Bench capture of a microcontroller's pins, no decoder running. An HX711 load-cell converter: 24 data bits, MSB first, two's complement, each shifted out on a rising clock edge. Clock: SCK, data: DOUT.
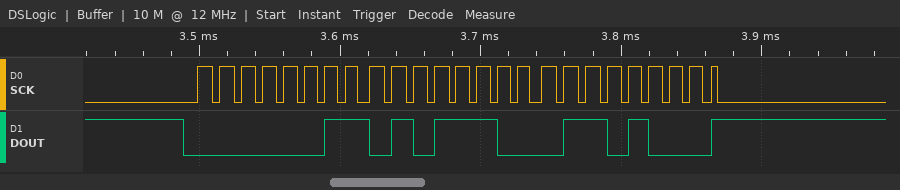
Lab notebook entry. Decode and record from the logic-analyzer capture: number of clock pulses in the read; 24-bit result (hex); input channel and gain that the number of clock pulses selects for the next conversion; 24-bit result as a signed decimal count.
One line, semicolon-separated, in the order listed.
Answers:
25; 0x035C68; channel A, gain 128; 220264
